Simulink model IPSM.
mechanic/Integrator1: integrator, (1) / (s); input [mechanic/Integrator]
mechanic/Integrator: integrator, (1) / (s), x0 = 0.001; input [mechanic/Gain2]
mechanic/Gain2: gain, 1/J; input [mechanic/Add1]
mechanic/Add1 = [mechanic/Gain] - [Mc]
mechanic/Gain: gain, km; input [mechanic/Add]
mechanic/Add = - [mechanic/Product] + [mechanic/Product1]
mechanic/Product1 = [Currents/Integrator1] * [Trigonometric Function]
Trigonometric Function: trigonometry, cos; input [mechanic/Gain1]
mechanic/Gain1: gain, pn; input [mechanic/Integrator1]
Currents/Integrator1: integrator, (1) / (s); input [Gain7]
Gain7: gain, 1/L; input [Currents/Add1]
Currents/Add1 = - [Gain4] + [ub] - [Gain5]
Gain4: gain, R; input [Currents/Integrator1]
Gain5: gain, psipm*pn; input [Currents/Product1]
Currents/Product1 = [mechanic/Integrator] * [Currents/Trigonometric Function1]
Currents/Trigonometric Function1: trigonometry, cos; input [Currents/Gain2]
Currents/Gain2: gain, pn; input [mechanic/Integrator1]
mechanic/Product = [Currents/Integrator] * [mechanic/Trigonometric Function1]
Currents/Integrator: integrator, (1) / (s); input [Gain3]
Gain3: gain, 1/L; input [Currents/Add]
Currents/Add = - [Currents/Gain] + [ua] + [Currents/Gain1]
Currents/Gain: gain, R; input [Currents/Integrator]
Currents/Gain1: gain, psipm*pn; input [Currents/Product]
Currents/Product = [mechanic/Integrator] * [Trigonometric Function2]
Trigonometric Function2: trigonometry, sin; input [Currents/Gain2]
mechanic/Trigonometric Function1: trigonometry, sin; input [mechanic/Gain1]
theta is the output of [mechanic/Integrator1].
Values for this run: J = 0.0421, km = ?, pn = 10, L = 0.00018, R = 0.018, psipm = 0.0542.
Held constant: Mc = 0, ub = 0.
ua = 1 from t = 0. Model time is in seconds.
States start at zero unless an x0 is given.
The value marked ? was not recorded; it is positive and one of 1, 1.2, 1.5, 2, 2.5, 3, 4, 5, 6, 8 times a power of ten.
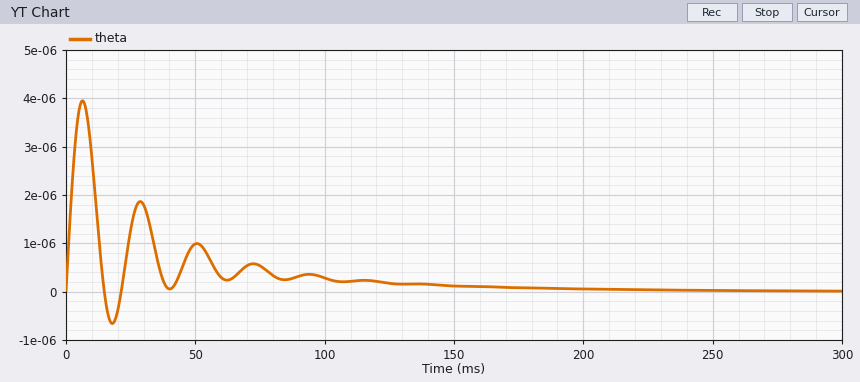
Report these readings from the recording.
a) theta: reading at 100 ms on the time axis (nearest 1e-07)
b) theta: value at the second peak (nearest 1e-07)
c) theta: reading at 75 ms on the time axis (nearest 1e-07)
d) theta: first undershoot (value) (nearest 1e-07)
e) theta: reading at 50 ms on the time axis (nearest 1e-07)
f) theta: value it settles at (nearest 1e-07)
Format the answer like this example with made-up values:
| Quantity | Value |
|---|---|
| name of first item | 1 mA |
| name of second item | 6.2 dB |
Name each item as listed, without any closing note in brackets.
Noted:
| Quantity | Value |
|---|---|
| theta: reading at 100 ms on the time axis | 0.0000003 |
| theta: value at the second peak | 0.0000019 |
| theta: reading at 75 ms on the time axis | 0.0000005 |
| theta: first undershoot (value) | -0.0000007 |
| theta: reading at 50 ms on the time axis | 0.0000010 |
| theta: value it settles at | 0.0000000 |
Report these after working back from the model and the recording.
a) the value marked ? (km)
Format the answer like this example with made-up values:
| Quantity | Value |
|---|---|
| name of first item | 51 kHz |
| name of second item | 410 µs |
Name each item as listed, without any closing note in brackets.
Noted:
| Quantity | Value |
|---|---|
| the value marked ? | 1 |
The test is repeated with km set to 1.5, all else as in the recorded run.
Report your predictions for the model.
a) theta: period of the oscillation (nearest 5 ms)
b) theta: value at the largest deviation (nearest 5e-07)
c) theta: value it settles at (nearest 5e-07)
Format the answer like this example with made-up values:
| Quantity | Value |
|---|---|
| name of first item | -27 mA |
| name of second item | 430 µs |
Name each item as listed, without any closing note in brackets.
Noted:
| Quantity | Value |
|---|---|
| theta: period of the oscillation | 20 ms |
| theta: value at the largest deviation | 0.0000030 |
| theta: value it settles at | 0.0000000 |
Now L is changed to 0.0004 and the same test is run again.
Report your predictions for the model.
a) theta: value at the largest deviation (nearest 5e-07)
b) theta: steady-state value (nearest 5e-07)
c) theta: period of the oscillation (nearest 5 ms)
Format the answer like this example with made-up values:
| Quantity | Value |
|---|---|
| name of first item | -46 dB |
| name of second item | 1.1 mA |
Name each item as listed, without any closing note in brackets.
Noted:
| Quantity | Value |
|---|---|
| theta: value at the largest deviation | 0.0000055 |
| theta: steady-state value | 0.0000000 |
| theta: period of the oscillation | 30 ms |
